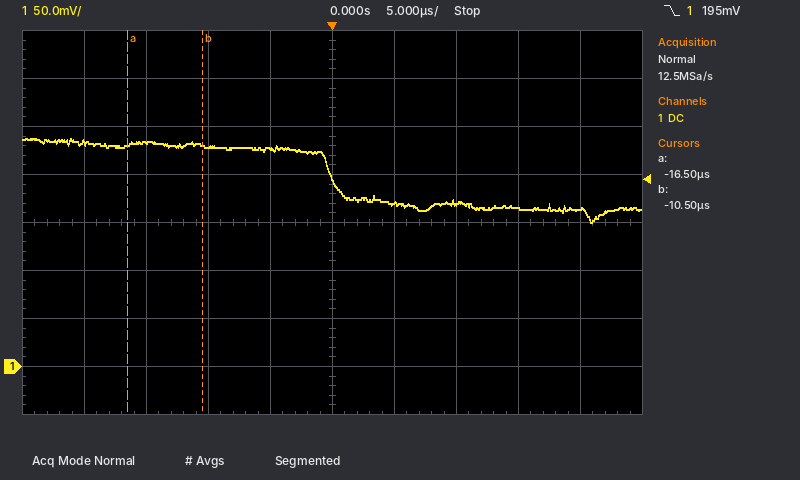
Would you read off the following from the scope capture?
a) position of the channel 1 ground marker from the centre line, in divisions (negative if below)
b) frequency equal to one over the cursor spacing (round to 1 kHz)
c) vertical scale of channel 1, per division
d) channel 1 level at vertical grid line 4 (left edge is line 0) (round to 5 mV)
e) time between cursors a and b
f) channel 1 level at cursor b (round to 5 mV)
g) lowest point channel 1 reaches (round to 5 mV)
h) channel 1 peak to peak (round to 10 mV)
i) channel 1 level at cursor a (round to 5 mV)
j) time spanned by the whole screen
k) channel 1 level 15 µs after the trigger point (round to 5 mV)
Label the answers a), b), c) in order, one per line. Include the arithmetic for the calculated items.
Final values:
a) -3.0 div
b) 1 / 6.0 µs ≈ 167 kHz
c) 50 mV
d) 225 mV
e) -10.5 µs − (-16.5 µs) = 6.0 µs
f) 230 mV
g) 150 mV
h) 90 mV
i) 230 mV
j) 50 µs
k) 165 mV
